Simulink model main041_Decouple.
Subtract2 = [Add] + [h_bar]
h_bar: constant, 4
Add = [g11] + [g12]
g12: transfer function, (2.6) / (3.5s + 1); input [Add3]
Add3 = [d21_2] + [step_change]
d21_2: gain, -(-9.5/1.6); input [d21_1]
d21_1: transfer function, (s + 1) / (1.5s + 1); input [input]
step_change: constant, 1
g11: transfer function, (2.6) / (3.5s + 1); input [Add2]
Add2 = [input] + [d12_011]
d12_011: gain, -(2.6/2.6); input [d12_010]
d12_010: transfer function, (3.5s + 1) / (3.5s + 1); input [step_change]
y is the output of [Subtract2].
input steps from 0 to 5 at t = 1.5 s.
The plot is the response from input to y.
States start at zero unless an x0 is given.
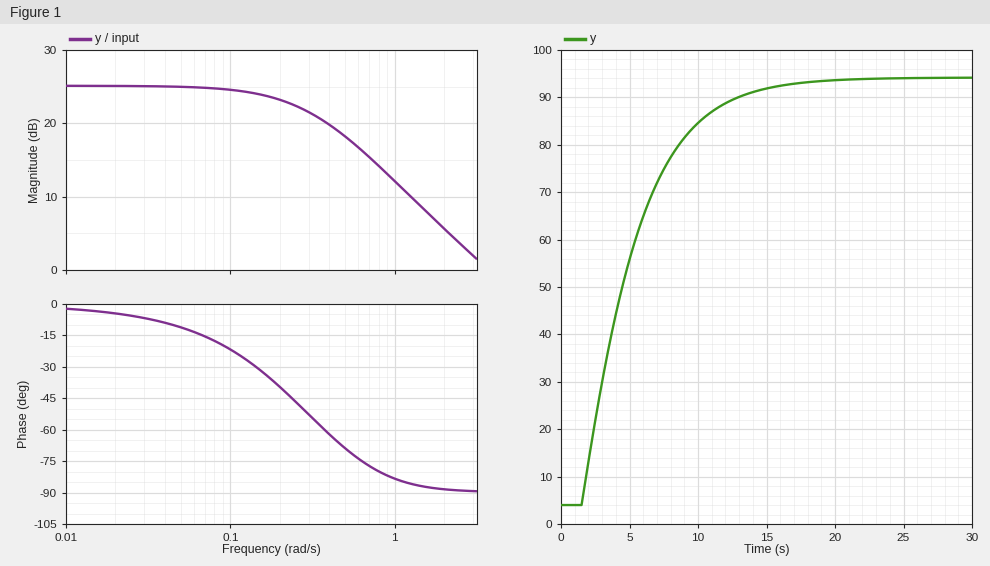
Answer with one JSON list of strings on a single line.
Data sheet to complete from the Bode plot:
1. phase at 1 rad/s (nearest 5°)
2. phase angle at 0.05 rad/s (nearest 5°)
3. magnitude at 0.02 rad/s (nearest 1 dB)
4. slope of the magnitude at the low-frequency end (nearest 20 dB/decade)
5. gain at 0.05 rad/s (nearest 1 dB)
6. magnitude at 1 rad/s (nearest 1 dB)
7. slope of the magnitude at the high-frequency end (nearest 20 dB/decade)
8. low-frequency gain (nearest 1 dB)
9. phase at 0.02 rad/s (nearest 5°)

["-85°", "-10°", "25 dB", "0 dB/decade", "25 dB", "12 dB", "-20 dB/decade", "25 dB", "-5°"]
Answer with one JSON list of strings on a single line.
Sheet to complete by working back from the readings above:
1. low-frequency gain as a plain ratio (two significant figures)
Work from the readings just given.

["18"]
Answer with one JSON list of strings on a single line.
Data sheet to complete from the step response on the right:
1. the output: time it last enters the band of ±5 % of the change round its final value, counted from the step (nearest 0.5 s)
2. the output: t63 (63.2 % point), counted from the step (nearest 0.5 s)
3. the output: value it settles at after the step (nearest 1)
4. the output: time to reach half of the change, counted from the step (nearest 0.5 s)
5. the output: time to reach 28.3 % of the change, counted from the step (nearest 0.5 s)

["11.0 s", "4.0 s", "94", "3.0 s", "1.5 s"]
